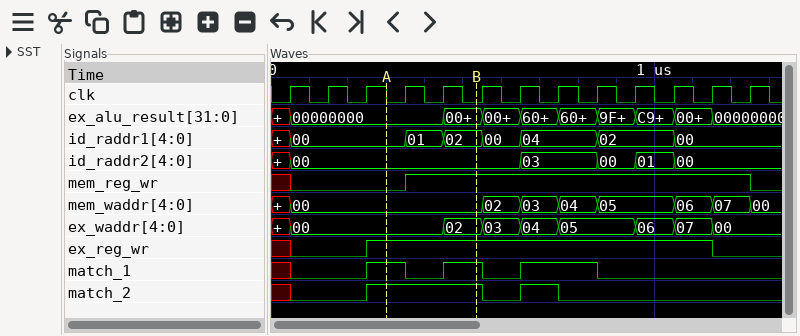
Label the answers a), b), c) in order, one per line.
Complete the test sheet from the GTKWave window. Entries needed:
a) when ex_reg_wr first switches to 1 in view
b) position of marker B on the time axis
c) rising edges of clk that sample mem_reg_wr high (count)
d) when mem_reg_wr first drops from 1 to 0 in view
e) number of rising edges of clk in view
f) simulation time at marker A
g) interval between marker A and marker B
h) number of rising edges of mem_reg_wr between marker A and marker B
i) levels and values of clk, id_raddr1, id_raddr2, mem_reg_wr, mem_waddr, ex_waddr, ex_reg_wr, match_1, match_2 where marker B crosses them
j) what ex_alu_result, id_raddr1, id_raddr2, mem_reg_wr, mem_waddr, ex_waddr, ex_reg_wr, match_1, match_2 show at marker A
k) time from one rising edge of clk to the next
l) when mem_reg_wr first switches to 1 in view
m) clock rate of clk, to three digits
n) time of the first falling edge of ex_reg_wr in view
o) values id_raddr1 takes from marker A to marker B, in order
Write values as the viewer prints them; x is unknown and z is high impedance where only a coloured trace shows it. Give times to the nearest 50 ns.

a) 250 ns
b) 550 ns
c) 9
d) 1250 ns
e) 13
f) 300 ns
g) 250 ns
h) 1
i) clk=0, id_raddr1=02, id_raddr2=00, mem_reg_wr=1, mem_waddr=00, ex_waddr=02, ex_reg_wr=1, match_1=1, match_2=1
j) ex_alu_result=00000000, id_raddr1=00, id_raddr2=00, mem_reg_wr=0, mem_waddr=00, ex_waddr=00, ex_reg_wr=1, match_1=1, match_2=1
k) 100 ns
l) 350 ns
m) 10.0 MHz
n) 1150 ns
o) 00, 01, 02
